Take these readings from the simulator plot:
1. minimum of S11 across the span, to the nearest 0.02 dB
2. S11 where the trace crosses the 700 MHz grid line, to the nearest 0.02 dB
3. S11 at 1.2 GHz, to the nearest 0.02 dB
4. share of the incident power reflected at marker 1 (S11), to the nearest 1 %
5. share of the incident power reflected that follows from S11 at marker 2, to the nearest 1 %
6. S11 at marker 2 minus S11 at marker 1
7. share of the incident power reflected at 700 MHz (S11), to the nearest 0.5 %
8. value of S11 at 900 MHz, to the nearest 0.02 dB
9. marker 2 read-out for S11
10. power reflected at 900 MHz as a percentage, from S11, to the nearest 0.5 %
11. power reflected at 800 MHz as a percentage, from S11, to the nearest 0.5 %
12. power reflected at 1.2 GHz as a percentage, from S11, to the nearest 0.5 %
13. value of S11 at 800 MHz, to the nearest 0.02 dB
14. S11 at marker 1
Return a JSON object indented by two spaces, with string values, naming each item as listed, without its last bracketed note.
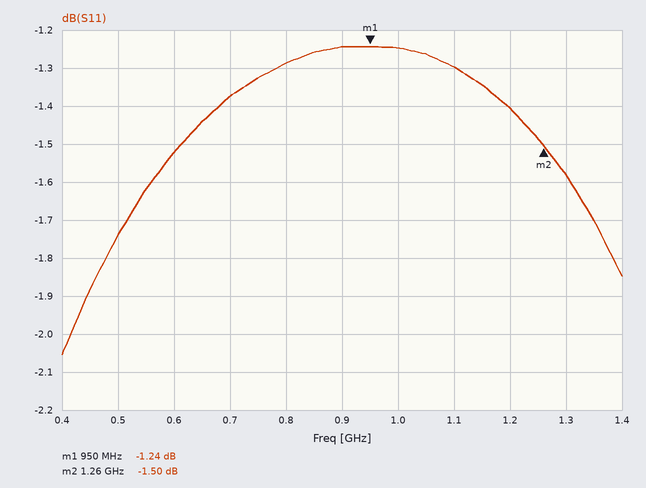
{
  "minimum of S11 across the span, to the nearest 0.02 dB": "-2.06 dB",
  "S11 where the trace crosses the 700 MHz grid line, to the nearest 0.02 dB": "-1.38 dB",
  "S11 at 1.2 GHz, to the nearest 0.02 dB": "-1.40 dB",
  "share of the incident power reflected at marker 1 (S11), to the nearest 1 %": "75 %",
  "share of the incident power reflected that follows from S11 at marker 2, to the nearest 1 %": "71 %",
  "S11 at marker 2 minus S11 at marker 1": "-0.26 dB",
  "share of the incident power reflected at 700 MHz (S11), to the nearest 0.5 %": "73.0 %",
  "value of S11 at 900 MHz, to the nearest 0.02 dB": "-1.24 dB",
  "marker 2 read-out for S11": "-1.50 dB",
  "power reflected at 900 MHz as a percentage, from S11, to the nearest 0.5 %": "75.0 %",
  "power reflected at 800 MHz as a percentage, from S11, to the nearest 0.5 %": "74.5 %",
  "power reflected at 1.2 GHz as a percentage, from S11, to the nearest 0.5 %": "72.5 %",
  "value of S11 at 800 MHz, to the nearest 0.02 dB": "-1.28 dB",
  "S11 at marker 1": "-1.24 dB"
}
